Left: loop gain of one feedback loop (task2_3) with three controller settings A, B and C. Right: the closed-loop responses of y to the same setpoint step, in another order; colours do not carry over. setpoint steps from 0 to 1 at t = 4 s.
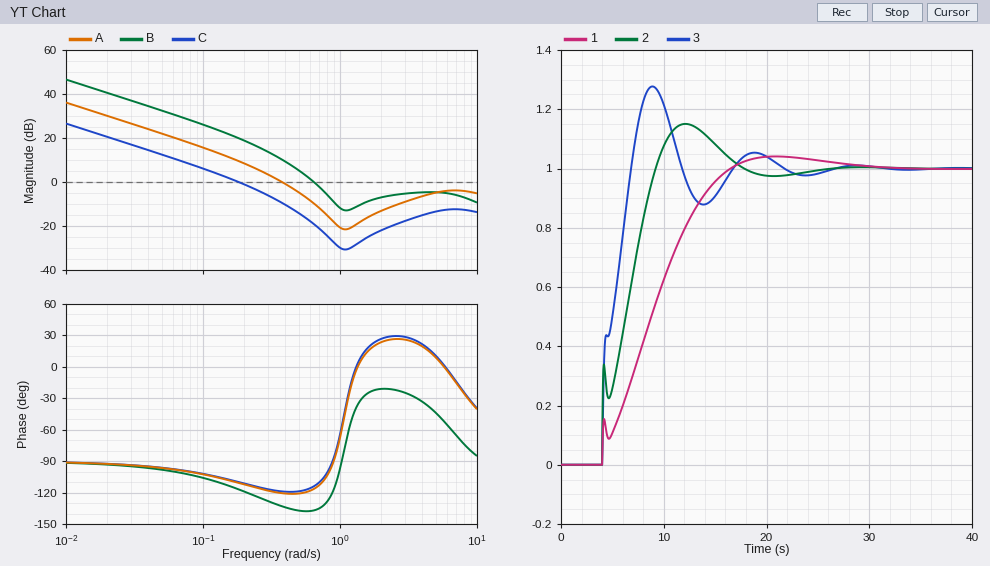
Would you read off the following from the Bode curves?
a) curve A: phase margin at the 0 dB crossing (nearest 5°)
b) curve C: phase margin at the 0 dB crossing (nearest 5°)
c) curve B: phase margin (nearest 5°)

60°
70°
45°
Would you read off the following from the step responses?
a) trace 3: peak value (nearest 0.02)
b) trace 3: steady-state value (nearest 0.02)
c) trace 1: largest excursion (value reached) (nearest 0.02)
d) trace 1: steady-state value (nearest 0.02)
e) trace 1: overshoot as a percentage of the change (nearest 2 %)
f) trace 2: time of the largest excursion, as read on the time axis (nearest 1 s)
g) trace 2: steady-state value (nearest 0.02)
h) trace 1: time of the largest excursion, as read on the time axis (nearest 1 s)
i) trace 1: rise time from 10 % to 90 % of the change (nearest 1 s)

1.28
1.00
1.04
1.00
4 %
12 s
1.00
21 s
10 s
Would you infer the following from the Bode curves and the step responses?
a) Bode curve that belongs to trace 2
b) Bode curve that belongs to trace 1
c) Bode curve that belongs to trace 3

A
C
B
